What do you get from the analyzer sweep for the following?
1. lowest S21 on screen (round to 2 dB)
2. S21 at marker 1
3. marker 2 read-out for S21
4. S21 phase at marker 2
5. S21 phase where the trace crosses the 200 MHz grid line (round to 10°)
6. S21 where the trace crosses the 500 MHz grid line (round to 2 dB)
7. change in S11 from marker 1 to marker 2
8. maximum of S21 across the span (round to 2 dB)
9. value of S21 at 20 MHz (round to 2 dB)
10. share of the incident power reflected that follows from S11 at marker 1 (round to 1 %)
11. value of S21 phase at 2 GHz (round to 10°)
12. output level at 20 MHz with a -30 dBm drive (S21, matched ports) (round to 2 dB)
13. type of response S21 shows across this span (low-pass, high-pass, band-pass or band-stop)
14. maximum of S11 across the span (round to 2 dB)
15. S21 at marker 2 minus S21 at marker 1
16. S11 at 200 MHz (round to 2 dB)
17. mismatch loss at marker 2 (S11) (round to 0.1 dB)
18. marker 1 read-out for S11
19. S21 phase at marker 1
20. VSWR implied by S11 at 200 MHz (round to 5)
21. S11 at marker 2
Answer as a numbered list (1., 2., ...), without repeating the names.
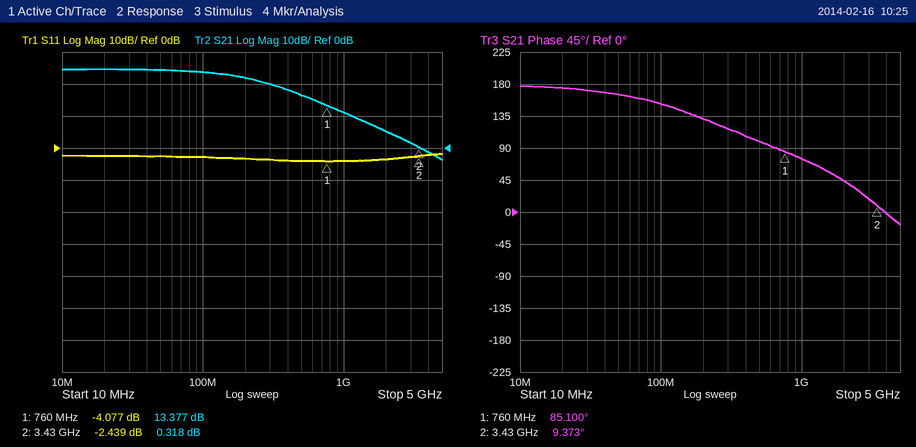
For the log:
1. -4 dB
2. 13.377 dB
3. 0.318 dB
4. 9.373°
5. 130°
6. 16 dB
7. 1.638 dB
8. 24 dB
9. 24 dB
10. 39 %
11. 40°
12. -6 dBm
13. low-pass
14. -2 dB
15. -13.059 dB
16. -4 dB
17. 3.7 dB
18. -4.077 dB
19. 85.100°
20. 5
21. -2.439 dB
